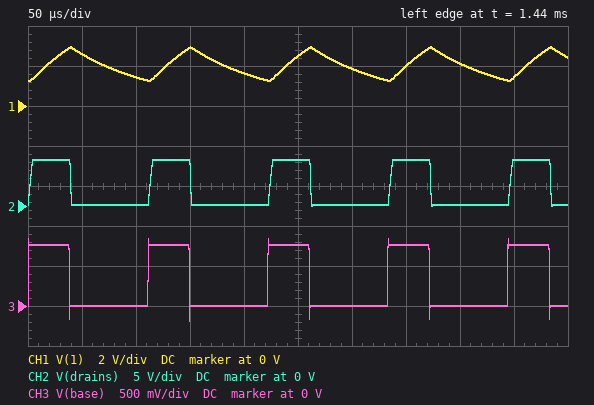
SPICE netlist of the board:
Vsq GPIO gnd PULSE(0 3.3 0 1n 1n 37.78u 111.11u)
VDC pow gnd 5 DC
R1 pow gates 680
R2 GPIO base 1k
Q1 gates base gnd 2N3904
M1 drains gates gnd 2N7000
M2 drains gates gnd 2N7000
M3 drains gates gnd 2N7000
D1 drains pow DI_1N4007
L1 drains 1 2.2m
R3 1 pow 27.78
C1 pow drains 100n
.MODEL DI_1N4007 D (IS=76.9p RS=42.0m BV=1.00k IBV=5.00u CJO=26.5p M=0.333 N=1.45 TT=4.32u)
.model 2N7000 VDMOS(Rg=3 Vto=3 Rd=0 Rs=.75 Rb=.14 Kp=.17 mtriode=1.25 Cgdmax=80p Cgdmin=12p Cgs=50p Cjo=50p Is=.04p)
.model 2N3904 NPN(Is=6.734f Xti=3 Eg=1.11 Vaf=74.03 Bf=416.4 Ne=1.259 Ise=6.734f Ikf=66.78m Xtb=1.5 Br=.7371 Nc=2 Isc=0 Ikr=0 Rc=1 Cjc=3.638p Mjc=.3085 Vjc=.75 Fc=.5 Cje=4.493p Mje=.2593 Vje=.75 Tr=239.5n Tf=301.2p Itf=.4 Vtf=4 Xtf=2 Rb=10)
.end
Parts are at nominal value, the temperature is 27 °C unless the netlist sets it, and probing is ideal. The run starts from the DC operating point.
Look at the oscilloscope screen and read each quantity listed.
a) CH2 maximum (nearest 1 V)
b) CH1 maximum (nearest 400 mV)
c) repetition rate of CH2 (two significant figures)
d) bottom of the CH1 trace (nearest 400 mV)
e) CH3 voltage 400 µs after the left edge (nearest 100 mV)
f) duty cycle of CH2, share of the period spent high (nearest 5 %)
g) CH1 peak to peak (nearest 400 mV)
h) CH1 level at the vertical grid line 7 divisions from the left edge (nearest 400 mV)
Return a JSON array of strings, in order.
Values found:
["6 V", "2.8 V", "9.0 kHz", "1.2 V", "0 V", "35 %", "1.6 V", "2.0 V"]
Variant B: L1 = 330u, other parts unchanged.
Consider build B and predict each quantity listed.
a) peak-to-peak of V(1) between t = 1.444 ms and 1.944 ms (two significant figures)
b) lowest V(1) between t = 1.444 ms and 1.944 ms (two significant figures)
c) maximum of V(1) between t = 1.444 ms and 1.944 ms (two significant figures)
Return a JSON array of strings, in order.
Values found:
["5.1 V", "200 mV", "5.3 V"]
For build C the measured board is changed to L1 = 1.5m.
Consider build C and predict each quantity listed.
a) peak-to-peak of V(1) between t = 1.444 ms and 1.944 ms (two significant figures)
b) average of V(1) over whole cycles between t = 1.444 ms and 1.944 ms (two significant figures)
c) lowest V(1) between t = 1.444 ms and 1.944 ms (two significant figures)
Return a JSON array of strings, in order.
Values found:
["2.4 V", "2.0 V", "980 mV"]
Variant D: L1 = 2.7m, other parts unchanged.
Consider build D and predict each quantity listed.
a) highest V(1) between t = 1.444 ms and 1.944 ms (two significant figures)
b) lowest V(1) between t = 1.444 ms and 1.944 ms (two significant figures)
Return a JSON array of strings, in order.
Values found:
["2.8 V", "1.4 V"]
